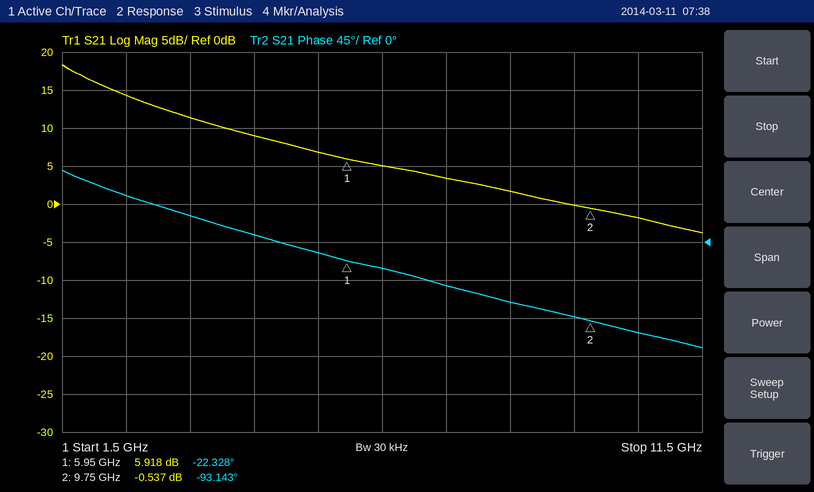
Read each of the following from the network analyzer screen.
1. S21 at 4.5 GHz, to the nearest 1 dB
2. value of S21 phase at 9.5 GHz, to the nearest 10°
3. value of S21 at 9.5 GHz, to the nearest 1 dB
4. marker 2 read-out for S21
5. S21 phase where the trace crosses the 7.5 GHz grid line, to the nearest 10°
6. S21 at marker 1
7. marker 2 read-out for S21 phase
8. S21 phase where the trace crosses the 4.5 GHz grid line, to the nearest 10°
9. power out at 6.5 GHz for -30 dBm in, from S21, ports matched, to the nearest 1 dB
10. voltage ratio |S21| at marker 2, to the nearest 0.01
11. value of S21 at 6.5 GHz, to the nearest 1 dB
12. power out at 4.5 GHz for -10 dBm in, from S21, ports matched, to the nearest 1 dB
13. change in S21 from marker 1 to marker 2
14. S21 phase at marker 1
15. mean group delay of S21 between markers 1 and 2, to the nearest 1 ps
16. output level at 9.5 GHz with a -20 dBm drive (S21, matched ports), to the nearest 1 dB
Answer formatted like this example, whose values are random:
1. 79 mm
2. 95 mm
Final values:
1. 9 dB
2. -90°
3. 0 dB
4. -0.537 dB
5. -50°
6. 5.918 dB
7. -93.143°
8. 10°
9. -25 dBm
10. 0.94
11. 5 dB
12. -1 dBm
13. -6.455 dB
14. -22.328°
15. 52 ps
16. -20 dBm
